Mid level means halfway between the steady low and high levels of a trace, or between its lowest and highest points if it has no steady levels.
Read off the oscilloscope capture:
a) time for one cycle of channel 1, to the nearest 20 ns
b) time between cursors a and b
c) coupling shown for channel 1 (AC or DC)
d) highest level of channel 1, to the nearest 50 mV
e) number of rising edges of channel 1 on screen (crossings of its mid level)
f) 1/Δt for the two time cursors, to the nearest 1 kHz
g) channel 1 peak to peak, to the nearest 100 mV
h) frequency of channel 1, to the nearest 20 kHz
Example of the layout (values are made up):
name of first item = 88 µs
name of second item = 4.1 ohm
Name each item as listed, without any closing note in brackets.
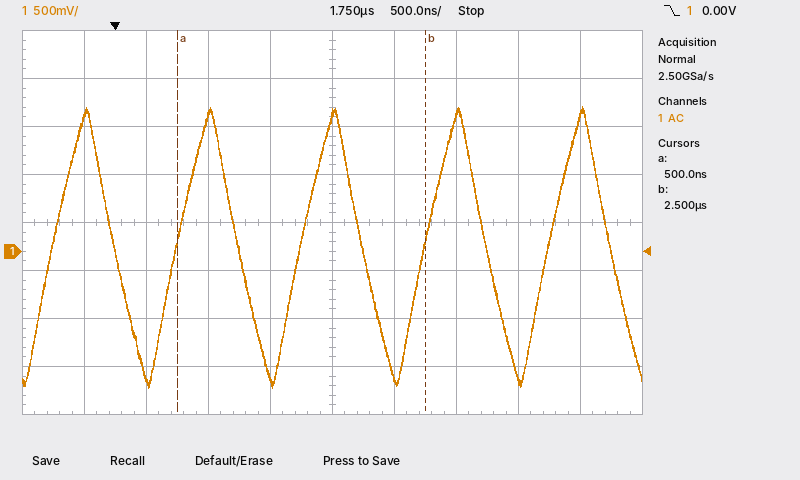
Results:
time for one cycle of channel 1, to the nearest 20 ns = 1.00 µs
time between cursors a and b = 2.00 µs
coupling shown for channel 1 = AC
highest level of channel 1, to the nearest 50 mV = 1.50 V
number of rising edges of channel 1 on screen = 5
1/Δt for the two time cursors, to the nearest 1 kHz = 500 kHz
channel 1 peak to peak, to the nearest 100 mV = 2.90 V
frequency of channel 1, to the nearest 20 kHz = 1.00 MHz
